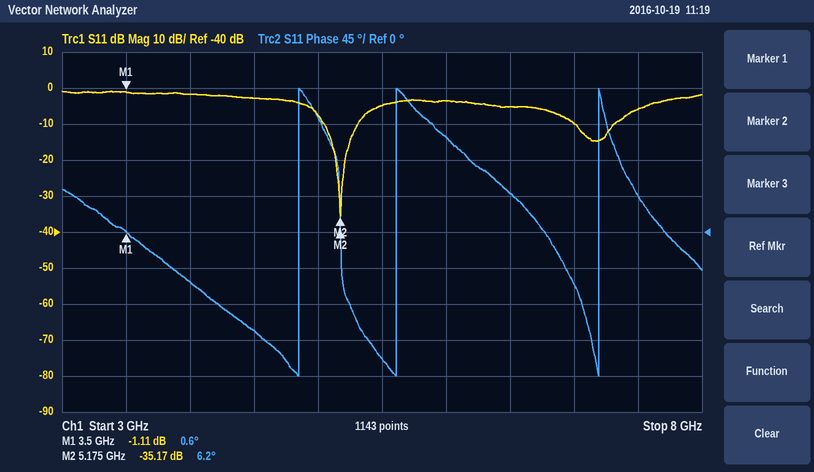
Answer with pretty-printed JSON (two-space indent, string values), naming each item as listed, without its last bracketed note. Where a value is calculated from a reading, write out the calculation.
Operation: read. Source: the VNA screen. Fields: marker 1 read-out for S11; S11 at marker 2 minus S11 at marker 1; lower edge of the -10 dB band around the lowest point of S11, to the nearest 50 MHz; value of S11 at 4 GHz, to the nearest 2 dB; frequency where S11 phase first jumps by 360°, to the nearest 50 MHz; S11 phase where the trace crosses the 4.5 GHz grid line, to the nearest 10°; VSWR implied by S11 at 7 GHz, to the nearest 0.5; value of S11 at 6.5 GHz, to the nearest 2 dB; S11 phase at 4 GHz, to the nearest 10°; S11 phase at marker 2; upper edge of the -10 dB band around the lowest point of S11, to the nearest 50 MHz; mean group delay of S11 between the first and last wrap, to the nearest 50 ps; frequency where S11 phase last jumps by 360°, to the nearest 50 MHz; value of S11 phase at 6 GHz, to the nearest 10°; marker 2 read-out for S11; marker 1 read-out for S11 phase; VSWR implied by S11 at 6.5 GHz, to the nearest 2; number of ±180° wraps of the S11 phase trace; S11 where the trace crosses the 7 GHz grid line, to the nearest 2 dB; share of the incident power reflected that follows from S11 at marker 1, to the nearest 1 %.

{
  "marker 1 read-out for S11": "-1.11 dB",
  "S11 at marker 2 minus S11 at marker 1": "-35.17 − (-1.11) = -34.06 dB",
  "lower edge of the -10 dB band around the lowest point of S11, to the nearest 50 MHz": "5.05 GHz",
  "value of S11 at 4 GHz, to the nearest 2 dB": "-2 dB",
  "frequency where S11 phase first jumps by 360°, to the nearest 50 MHz": "4.85 GHz",
  "S11 phase where the trace crosses the 4.5 GHz grid line, to the nearest 10°": "-120°",
  "VSWR implied by S11 at 7 GHz, to the nearest 0.5": "|Γ| = 10^(-10/20) = 0.3162; VSWR = (1 + 0.3162)/(1 − 0.3162) ≈ 1.92, so 2.0 to the nearest 0.5",
  "value of S11 at 6.5 GHz, to the nearest 2 dB": "-6 dB",
  "S11 phase at 4 GHz, to the nearest 10°": "-60°",
  "S11 phase at marker 2": "6.2°",
  "upper edge of the -10 dB band around the lowest point of S11, to the nearest 50 MHz": "5.30 GHz",
  "mean group delay of S11 between the first and last wrap, to the nearest 50 ps": "2 cycles / (7.20 GHz − 4.85 GHz) ≈ 851 ps, so 850 ps to the nearest 50 ps",
  "frequency where S11 phase last jumps by 360°, to the nearest 50 MHz": "7.20 GHz",
  "value of S11 phase at 6 GHz, to the nearest 10°": "120°",
  "marker 2 read-out for S11": "-35.17 dB",
  "marker 1 read-out for S11 phase": "0.6°",
  "VSWR implied by S11 at 6.5 GHz, to the nearest 2": "|Γ| = 10^(-6/20) = 0.5012; VSWR = (1 + 0.5012)/(1 − 0.5012) ≈ 3.01, so 4 to the nearest 2",
  "number of ±180° wraps of the S11 phase trace": "3",
  "S11 where the trace crosses the 7 GHz grid line, to the nearest 2 dB": "-10 dB",
  "share of the incident power reflected that follows from S11 at marker 1, to the nearest 1 %": "10^(-1.11/10) ≈ 77 %"
}
